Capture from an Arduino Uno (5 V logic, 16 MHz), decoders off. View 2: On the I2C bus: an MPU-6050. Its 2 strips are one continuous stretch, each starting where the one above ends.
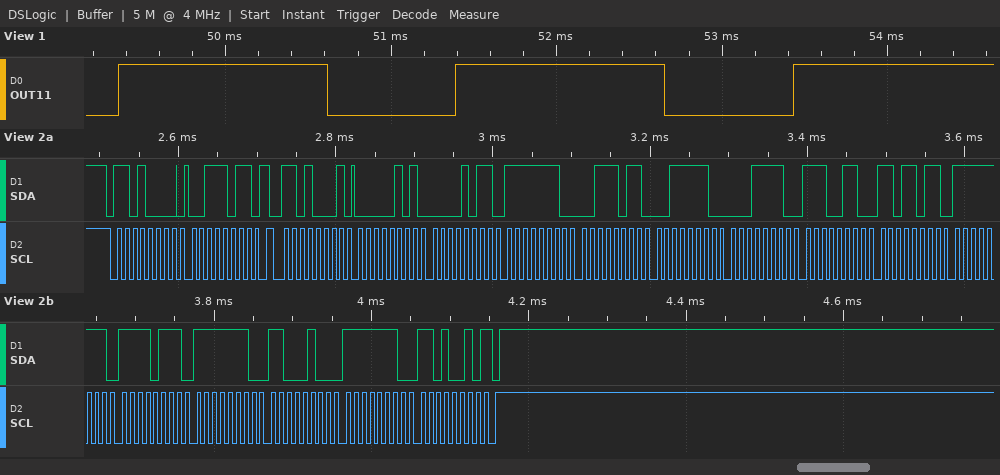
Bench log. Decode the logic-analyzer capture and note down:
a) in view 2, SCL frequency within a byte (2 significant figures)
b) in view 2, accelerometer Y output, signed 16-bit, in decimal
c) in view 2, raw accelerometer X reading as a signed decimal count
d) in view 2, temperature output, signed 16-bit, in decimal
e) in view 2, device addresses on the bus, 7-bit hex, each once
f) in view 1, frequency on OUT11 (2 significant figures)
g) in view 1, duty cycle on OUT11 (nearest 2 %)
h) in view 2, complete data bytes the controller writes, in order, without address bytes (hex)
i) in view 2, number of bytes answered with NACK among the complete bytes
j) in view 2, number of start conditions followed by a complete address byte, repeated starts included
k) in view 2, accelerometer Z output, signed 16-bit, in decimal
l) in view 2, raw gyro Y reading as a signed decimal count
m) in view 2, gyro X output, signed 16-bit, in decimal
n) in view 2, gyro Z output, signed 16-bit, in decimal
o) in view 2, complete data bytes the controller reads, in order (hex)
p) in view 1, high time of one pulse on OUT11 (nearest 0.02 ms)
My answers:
100 kHz
-453
1291
-6437
0x68
490 Hz
62 %
3B
1
2
15902
-316
-9
-302
05 0B FE 3B 3E 1E E6 DB FF F7 FE C4 FE D2
1.26 ms
